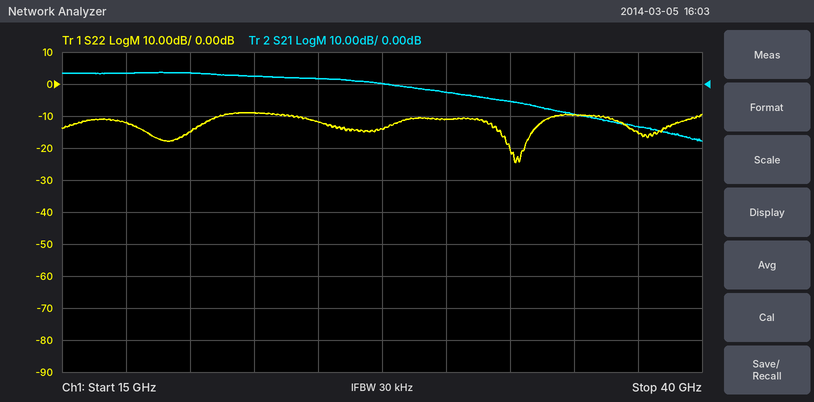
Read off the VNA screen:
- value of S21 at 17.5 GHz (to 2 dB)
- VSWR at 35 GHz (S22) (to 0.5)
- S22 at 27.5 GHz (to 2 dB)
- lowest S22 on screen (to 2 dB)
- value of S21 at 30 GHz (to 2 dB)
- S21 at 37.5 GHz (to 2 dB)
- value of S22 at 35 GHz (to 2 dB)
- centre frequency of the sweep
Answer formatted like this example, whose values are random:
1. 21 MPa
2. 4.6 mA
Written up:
1. 4 dB
2. 2.0
3. -14 dB
4. -24 dB
5. -2 dB
6. -14 dB
7. -10 dB
8. 27.5 GHz
